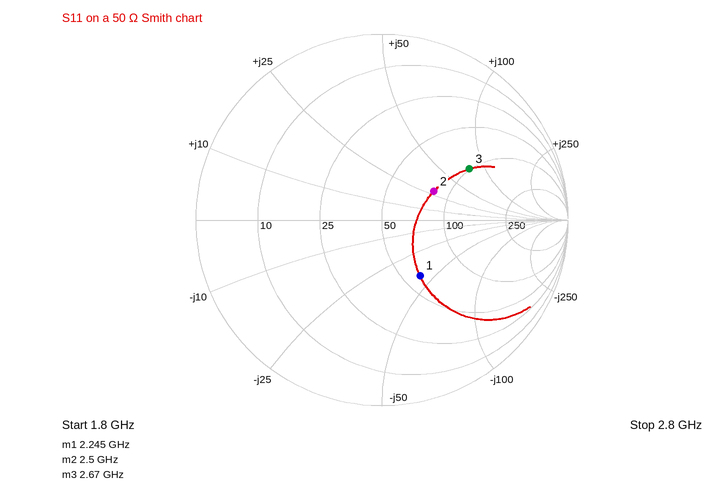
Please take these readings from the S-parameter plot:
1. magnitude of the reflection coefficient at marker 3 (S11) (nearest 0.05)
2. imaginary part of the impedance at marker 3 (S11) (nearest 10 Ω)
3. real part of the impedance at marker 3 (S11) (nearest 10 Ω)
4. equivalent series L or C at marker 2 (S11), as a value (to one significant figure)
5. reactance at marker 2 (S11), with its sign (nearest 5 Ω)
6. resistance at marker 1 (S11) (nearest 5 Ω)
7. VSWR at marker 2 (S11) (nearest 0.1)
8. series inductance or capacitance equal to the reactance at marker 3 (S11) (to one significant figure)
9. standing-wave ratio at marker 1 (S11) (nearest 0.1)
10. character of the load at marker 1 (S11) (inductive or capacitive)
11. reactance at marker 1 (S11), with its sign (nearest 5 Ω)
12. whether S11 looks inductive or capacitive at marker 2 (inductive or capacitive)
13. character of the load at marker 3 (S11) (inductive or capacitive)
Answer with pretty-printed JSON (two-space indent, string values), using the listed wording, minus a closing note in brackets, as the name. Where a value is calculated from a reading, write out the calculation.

{
  "magnitude of the reflection coefficient at marker 3 (S11)": "0.55",
  "imaginary part of the impedance at marker 3 (S11)": "+80 Ω",
  "real part of the impedance at marker 3 (S11)": "100 Ω",
  "equivalent series L or C at marker 2 (S11), as a value": "L = 30 Ω/(2π × 2.5 GHz) ≈ 2 nH",
  "reactance at marker 2 (S11), with its sign": "+30 Ω",
  "resistance at marker 1 (S11)": "60 Ω",
  "VSWR at marker 2 (S11)": "1.9",
  "series inductance or capacitance equal to the reactance at marker 3 (S11)": "L = 80 Ω/(2π × 2.67 GHz) ≈ 5 nH",
  "standing-wave ratio at marker 1 (S11)": "2.1",
  "character of the load at marker 1 (S11)": "capacitive",
  "reactance at marker 1 (S11), with its sign": "-40 Ω",
  "whether S11 looks inductive or capacitive at marker 2": "inductive",
  "character of the load at marker 3 (S11)": "inductive"
}
